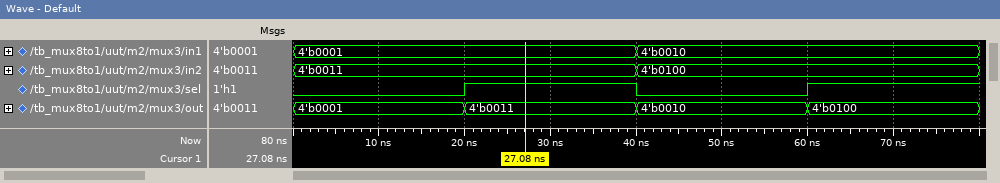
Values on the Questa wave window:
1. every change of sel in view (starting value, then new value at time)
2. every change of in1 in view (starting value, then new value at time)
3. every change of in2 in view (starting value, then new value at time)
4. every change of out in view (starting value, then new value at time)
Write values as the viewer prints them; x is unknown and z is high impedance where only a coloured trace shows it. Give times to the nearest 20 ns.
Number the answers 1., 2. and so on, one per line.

1. 0, 1 at 20 ns, 0 at 40 ns, 1 at 60 ns
2. 4'b0001, 4'b0010 at 40 ns
3. 4'b0011, 4'b0100 at 40 ns
4. 4'b0001, 4'b0011 at 20 ns, 4'b0010 at 40 ns, 4'b0100 at 60 ns
